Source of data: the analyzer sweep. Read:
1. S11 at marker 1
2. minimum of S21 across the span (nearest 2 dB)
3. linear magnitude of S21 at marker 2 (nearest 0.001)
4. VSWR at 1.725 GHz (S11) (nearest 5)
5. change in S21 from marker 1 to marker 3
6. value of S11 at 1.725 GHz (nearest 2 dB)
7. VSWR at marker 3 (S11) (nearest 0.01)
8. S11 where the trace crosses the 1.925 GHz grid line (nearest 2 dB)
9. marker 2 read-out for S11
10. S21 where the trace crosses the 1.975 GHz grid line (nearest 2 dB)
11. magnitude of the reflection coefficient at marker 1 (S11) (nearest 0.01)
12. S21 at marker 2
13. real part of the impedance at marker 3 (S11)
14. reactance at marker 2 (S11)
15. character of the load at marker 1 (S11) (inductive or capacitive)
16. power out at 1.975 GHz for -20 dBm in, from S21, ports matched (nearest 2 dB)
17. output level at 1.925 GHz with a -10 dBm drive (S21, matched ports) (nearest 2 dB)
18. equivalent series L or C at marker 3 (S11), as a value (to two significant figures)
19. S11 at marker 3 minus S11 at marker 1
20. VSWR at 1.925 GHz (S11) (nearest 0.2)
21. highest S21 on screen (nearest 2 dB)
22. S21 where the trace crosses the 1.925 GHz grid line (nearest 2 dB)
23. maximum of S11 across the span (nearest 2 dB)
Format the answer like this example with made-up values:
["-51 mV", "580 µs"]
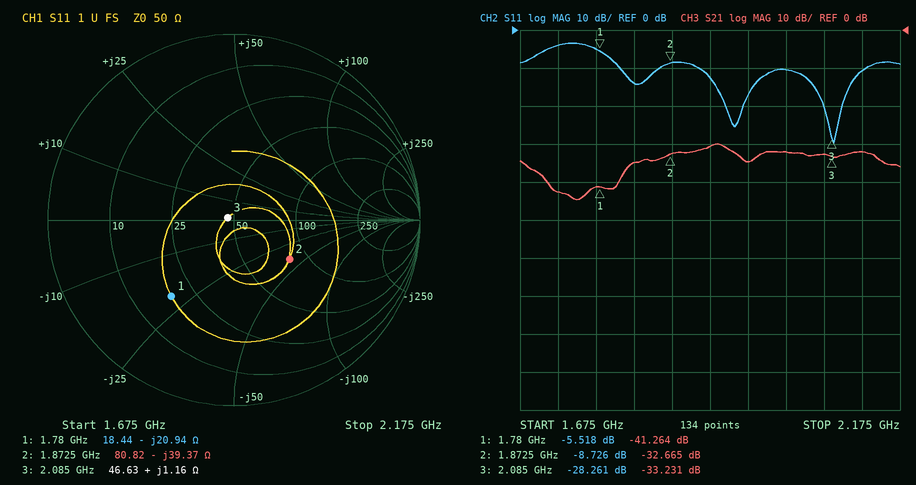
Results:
["-5.518 dB", "-44 dB", "0.023", "5", "8.033 dB", "-4 dB", "1.08", "-12 dB", "-8.726 dB", "-34 dB", "0.53", "-32.665 dB", "46.63 Ω", "-39.37 Ω", "capacitive", "-54 dBm", "-40 dBm", "89 pH", "-22.743 dB", "1.6", "-30 dB", "-30 dB", "-4 dB"]
